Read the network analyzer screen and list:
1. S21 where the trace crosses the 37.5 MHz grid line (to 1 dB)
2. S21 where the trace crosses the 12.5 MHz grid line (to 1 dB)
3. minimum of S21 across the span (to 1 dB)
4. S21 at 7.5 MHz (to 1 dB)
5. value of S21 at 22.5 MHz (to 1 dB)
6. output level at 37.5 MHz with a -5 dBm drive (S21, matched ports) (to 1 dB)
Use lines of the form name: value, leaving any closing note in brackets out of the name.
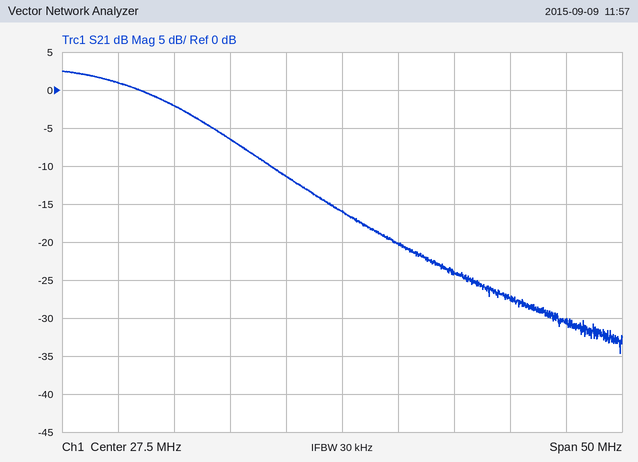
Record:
S21 where the trace crosses the 37.5 MHz grid line: -24 dB
S21 where the trace crosses the 12.5 MHz grid line: -2 dB
minimum of S21 across the span: -35 dB
S21 at 7.5 MHz: 1 dB
value of S21 at 22.5 MHz: -11 dB
output level at 37.5 MHz with a -5 dBm drive (S21, matched ports): -29 dBm
